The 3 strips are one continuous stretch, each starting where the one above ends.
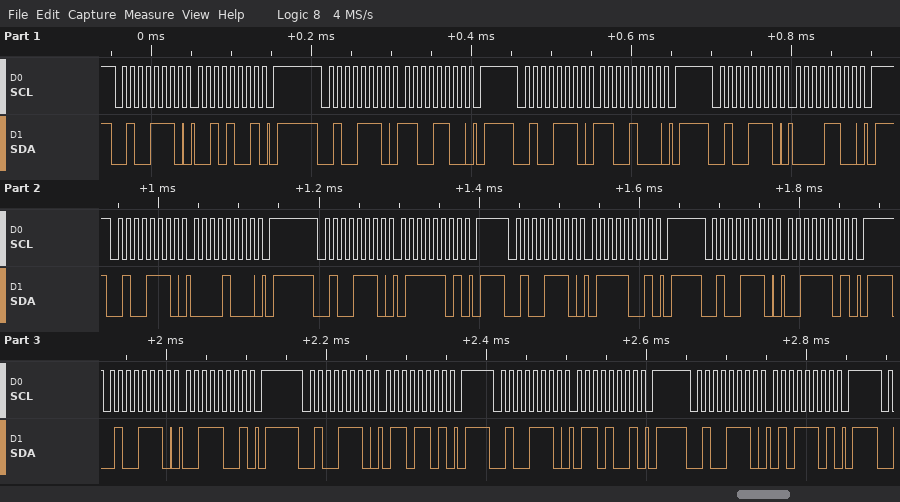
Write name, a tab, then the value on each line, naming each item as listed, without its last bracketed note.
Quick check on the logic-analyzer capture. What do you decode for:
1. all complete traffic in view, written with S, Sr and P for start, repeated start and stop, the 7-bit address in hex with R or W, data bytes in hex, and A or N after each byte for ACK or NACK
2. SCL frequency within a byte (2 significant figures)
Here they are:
all complete traffic in view, written with S, Sr and P for start, repeated start and stop, the 7-bit address in hex with R or W, data bytes in hex, and A or N after each byte for ACK or NACK	S 27W A 29 A P S 27W A CC A P S 27W A C8 A P S 27W A 0C A P S 27W A 08 A P S 27W A 7D A P S 27W A 79 A P S 27W A 3D A P S 27W A 39 A P S 27W A 6D A P S 27W A 69 A P S 27W A 5D A P
SCL frequency within a byte	100 kHz
